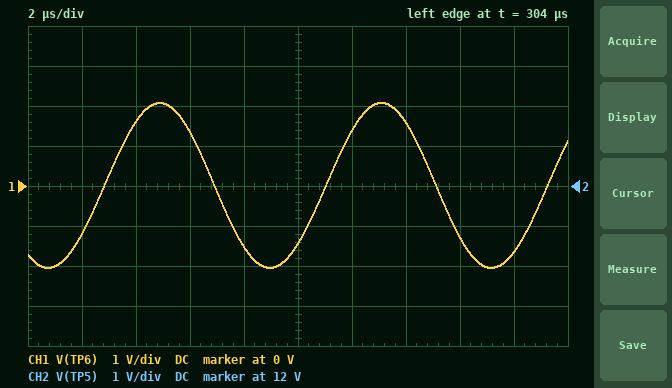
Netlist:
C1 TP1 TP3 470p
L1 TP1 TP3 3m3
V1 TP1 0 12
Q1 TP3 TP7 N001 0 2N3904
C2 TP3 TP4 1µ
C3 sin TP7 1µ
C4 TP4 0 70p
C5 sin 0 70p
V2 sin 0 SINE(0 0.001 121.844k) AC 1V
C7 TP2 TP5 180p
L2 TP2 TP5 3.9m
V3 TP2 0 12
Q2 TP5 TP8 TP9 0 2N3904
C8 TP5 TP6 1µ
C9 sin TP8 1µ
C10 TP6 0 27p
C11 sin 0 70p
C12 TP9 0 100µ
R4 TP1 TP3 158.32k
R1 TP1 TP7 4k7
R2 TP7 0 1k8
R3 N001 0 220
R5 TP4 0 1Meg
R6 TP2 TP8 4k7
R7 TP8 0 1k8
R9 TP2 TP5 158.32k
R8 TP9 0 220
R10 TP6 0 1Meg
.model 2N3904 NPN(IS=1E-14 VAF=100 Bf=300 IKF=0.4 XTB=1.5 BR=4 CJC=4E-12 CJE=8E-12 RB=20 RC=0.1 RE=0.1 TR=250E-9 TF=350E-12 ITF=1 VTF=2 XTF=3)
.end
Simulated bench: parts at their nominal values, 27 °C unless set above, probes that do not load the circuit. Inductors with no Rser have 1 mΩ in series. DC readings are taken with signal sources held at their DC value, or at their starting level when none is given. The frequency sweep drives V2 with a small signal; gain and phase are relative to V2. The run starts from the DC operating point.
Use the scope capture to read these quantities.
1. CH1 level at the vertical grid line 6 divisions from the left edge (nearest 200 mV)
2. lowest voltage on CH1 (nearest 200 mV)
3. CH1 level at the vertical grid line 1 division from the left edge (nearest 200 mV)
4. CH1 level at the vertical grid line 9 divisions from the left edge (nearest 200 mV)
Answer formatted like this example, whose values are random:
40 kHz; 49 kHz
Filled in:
1.4 V; -2.0 V; -1.2 V; -1.6 V
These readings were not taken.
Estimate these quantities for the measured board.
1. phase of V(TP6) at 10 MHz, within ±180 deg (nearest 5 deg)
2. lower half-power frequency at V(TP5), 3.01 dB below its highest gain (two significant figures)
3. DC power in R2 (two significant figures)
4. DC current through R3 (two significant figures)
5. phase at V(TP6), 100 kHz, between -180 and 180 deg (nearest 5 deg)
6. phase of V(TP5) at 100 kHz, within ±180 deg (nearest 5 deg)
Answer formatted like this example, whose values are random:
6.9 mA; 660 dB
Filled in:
80 deg; 140 kHz; 6.0 mW; 12 mA; -110 deg; -110 deg
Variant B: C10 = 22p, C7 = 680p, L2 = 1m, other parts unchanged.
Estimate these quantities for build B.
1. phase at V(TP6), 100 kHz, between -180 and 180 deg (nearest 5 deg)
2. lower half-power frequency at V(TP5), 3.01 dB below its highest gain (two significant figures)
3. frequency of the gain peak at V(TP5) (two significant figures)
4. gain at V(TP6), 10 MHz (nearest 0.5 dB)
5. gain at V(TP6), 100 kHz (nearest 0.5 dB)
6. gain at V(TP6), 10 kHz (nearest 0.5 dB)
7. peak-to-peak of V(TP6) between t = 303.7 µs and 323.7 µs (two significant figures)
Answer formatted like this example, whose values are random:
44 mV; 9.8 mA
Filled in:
-95 deg; 180 kHz; 190 kHz; 19.0 dB; 51.0 dB; 28.0 dB; 1.1 V
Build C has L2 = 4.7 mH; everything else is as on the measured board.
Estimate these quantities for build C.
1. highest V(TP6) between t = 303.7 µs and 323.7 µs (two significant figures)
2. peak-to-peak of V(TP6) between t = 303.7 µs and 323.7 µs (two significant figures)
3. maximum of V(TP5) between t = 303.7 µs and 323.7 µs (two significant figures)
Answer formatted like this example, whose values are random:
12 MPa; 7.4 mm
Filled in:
2.7 V; 5.3 V; 15 V
